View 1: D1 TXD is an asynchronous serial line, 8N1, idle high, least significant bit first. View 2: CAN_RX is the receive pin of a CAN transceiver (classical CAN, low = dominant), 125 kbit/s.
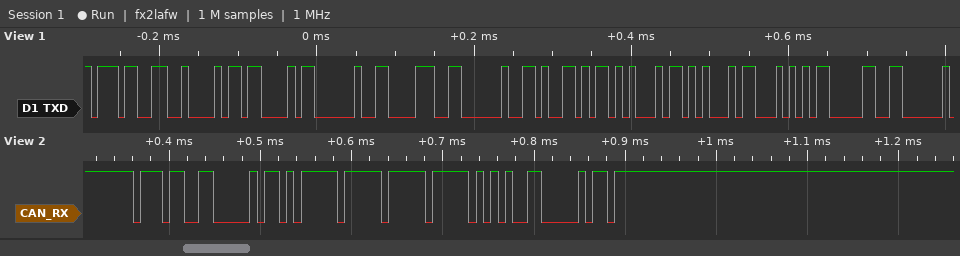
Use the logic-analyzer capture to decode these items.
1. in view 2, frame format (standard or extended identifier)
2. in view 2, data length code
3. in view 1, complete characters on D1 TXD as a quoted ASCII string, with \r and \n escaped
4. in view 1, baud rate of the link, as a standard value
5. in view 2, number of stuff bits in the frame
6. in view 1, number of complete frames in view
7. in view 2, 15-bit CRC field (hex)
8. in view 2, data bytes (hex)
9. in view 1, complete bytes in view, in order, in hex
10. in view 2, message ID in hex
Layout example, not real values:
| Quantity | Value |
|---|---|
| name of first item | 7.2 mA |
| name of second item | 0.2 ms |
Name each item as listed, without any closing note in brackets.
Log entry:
| Quantity | Value |
|---|---|
| in view 2, frame format | standard |
| in view 2, data length code | 3 |
| in view 1, complete characters on D1 TXD as a quoted ASCII string, with \r and \n escaped | "7BC 8 YEET0" |
| in view 1, baud rate of the link, as a standard value | 115200 baud |
| in view 2, number of stuff bits in the frame | 6 |
| in view 1, number of complete frames in view | 11 |
| in view 2, 15-bit CRC field | 0x2981 |
| in view 2, data bytes | 5F FF FF |
| in view 1, complete bytes in view, in order, in hex | 37 42 43 20 38 20 59 45 45 54 30 |
| in view 2, message ID in hex | 0x766 |
